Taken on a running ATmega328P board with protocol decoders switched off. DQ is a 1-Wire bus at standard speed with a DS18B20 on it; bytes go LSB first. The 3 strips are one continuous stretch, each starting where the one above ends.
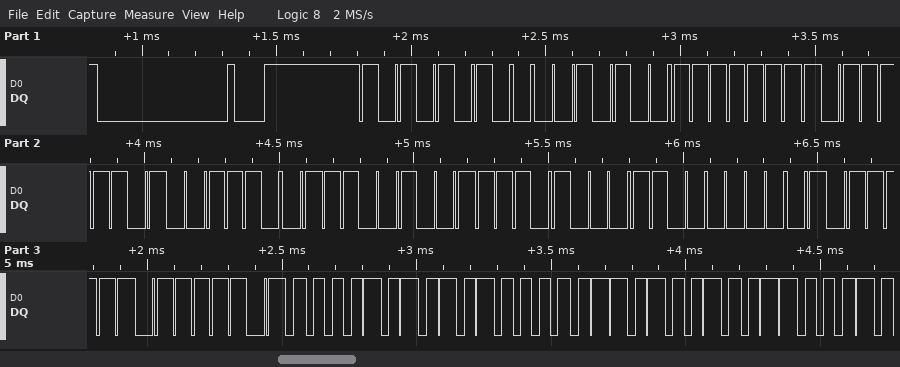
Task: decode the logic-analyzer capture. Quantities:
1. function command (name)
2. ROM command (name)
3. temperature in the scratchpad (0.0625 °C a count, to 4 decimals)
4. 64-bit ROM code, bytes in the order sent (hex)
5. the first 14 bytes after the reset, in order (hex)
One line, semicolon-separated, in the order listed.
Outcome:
Read Scratchpad; Match ROM; 85.0000 °C; 28 FF BE 9C 93 17 03 FA; 55 28 FF BE 9C 93 17 03 FA BE 50 05 4B 46
